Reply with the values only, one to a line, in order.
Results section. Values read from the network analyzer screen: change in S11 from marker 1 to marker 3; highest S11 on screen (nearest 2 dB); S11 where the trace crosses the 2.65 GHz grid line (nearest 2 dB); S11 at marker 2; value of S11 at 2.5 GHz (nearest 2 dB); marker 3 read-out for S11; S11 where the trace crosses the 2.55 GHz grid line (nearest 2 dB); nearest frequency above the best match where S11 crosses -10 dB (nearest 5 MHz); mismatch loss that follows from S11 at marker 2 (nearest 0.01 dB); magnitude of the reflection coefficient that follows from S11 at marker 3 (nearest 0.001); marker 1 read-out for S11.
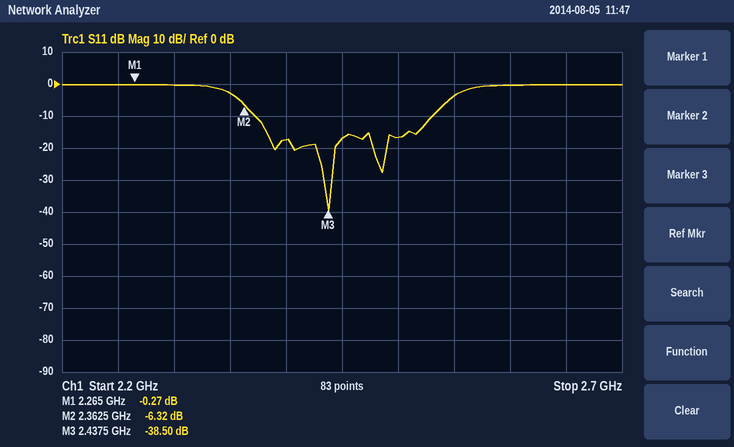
-38.23 dB
0 dB
0 dB
-6.32 dB
-16 dB
-38.50 dB
-4 dB
2.530 GHz
1.15 dB
0.012
-0.27 dB
